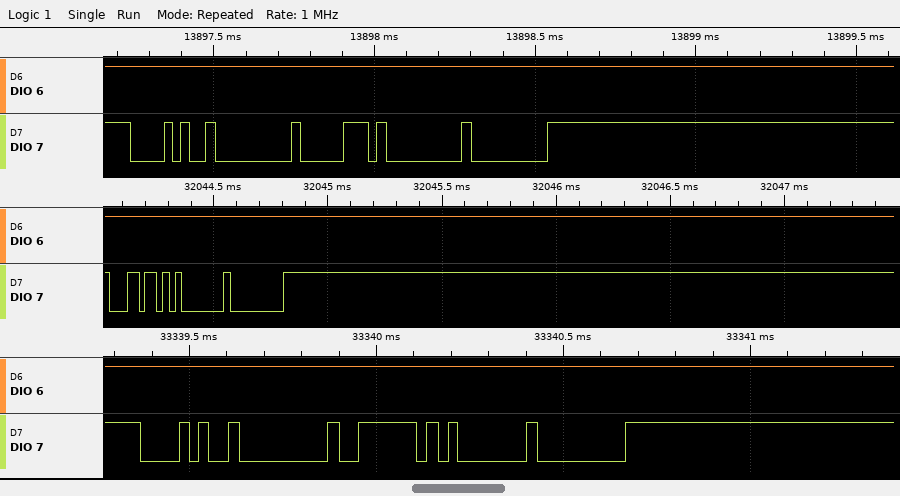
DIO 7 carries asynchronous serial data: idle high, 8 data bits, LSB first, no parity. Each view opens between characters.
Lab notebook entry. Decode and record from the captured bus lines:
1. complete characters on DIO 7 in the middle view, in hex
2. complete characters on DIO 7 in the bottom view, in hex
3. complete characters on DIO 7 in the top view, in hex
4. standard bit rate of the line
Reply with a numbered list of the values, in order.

1. 6C, 01, 00
2. 28, 00, 7E, 01, 00
3. 28, 00, 70, 00, 00
4. 38400 baud
